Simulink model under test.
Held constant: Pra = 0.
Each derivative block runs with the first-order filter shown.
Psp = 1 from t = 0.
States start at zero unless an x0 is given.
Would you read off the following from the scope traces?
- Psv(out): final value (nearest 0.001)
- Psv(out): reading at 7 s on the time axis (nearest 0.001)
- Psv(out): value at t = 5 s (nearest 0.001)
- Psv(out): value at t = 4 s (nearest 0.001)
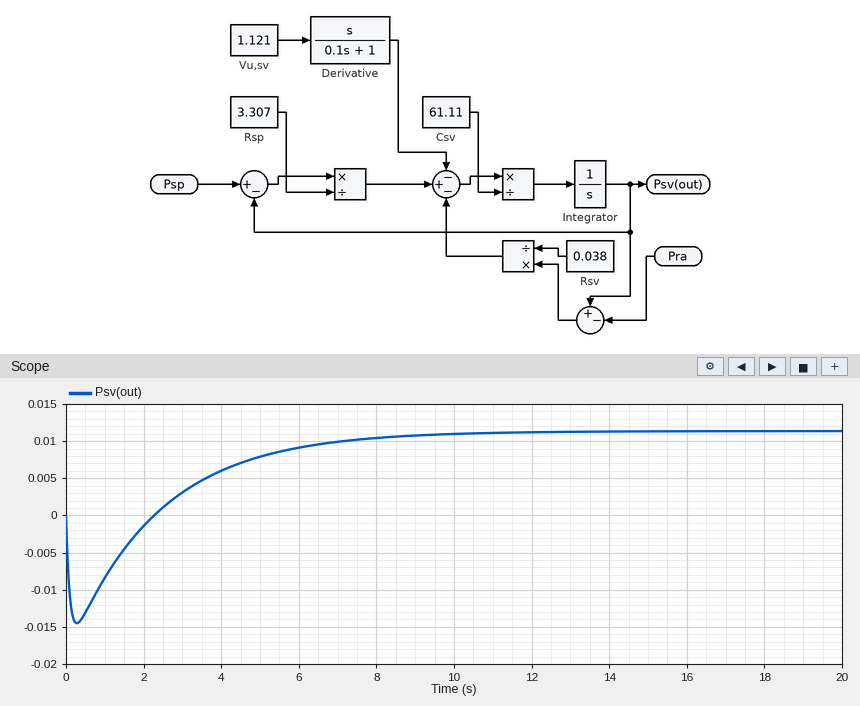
0.011
0.010
0.008
0.006
